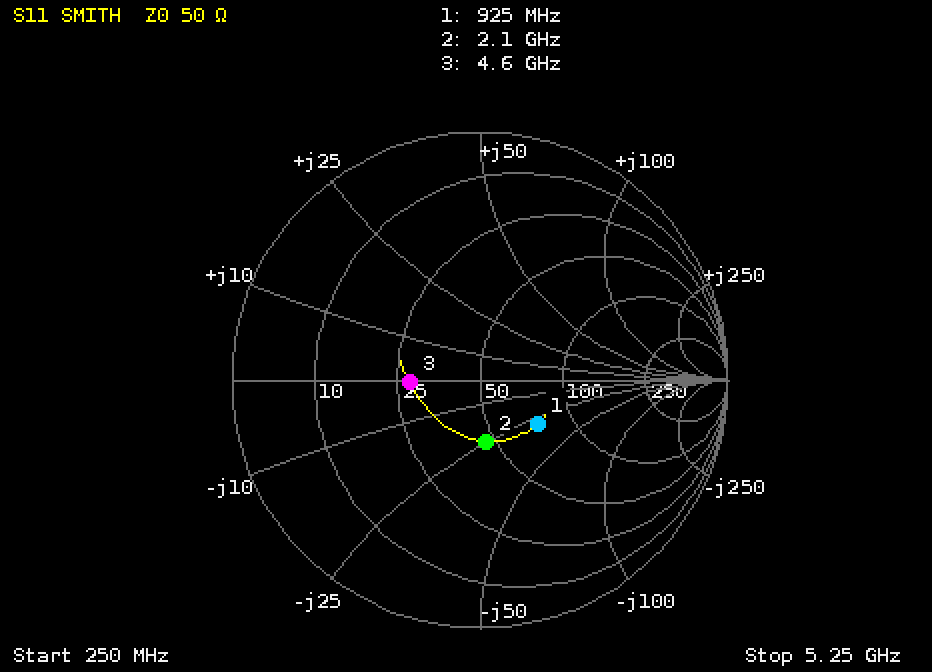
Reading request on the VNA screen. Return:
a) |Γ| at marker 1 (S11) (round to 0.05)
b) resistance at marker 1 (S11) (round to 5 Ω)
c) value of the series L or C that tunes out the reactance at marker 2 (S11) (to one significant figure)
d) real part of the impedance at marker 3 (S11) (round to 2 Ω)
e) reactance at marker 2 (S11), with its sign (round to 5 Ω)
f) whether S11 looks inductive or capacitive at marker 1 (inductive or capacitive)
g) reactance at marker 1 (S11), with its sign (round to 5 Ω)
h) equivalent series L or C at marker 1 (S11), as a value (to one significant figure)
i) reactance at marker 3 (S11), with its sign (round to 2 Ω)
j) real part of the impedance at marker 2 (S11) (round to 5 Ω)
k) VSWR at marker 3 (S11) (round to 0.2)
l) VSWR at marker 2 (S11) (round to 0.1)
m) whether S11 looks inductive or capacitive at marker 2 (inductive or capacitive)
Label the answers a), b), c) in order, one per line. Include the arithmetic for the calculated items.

a) 0.30
b) 75 Ω
c) L = 25 Ω/(2π × 2.1 GHz) ≈ 2 nH
d) 28 Ω
e) -25 Ω
f) capacitive
g) -30 Ω
h) C = 1/(2π × 925 MHz × 30 Ω) ≈ 6 pF
i) 0 Ω
j) 45 Ω
k) 1.8
l) 1.7
m) capacitive
